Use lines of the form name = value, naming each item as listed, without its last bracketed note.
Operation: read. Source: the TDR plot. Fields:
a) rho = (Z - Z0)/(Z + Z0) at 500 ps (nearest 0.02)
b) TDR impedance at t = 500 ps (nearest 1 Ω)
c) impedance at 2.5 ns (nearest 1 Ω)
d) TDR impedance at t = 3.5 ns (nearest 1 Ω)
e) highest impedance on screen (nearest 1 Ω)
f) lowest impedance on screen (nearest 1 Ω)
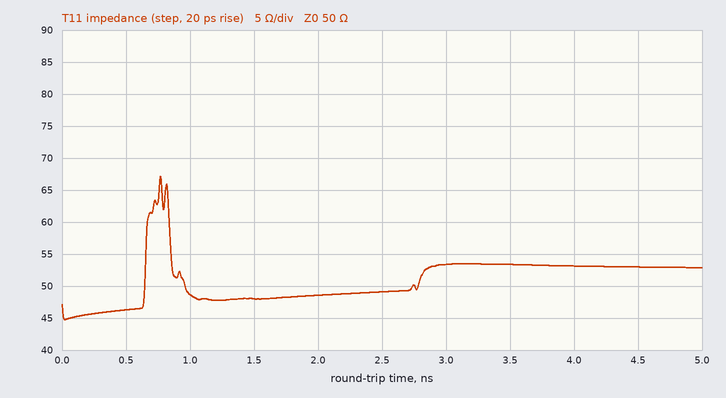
rho = (Z - Z0)/(Z + Z0) at 500 ps = -0.04
TDR impedance at t = 500 ps = 46 Ω
impedance at 2.5 ns = 49 Ω
TDR impedance at t = 3.5 ns = 53 Ω
highest impedance on screen = 67 Ω
lowest impedance on screen = 45 Ω
